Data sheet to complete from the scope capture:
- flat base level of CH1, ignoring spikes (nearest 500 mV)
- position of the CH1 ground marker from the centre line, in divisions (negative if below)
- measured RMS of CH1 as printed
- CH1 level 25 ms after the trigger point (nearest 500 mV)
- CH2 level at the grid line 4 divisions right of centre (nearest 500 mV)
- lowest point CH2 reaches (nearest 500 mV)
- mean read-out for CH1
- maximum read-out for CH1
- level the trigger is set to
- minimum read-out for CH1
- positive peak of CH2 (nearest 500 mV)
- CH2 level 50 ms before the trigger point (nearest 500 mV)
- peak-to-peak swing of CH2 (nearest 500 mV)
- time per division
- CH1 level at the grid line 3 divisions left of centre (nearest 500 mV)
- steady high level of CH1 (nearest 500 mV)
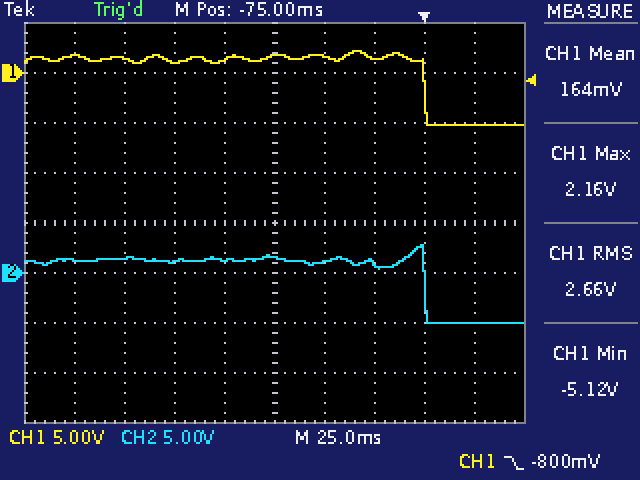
-5.0 V
+3.0 div
2.66 V
-5.0 V
-5.0 V
-5.0 V
164 mV
2.16 V
-800 mV
-5.12 V
3.0 V
1.0 V
8.0 V
25 ms
1.5 V
1.5 V
